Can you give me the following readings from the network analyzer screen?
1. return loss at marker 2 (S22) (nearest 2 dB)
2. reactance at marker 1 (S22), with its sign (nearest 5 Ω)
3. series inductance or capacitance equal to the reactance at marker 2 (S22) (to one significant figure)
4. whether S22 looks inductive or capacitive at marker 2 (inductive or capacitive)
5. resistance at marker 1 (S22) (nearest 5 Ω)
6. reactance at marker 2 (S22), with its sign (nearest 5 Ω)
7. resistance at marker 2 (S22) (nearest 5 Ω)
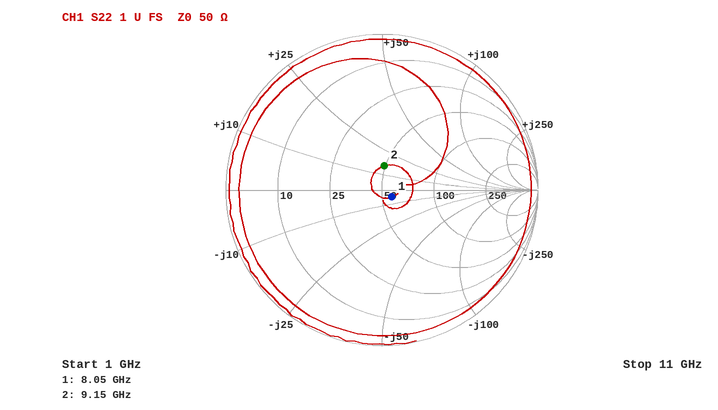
16 dB
-5 Ω
300 pH
inductive
55 Ω
+15 Ω
50 Ω
